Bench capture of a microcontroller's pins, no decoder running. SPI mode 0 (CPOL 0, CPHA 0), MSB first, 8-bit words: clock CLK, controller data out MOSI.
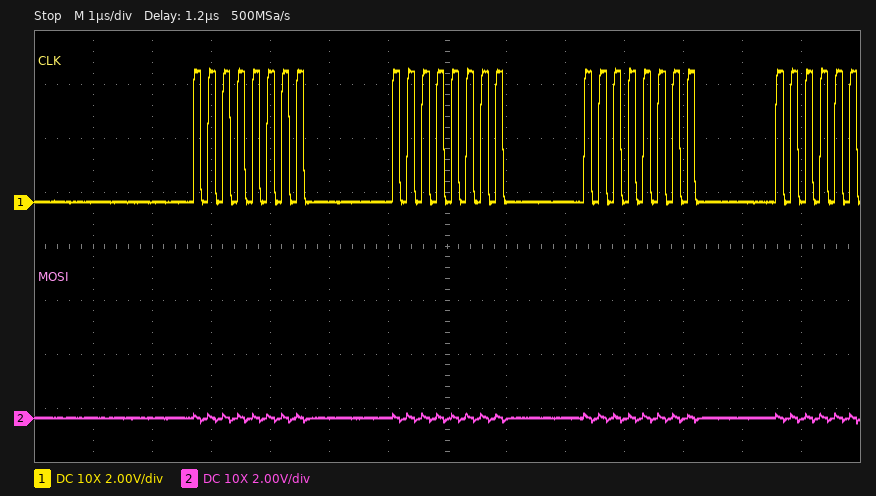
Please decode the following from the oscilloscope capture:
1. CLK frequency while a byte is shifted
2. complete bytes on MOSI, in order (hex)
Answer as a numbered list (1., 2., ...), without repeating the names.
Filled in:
1. 4 MHz
2. 00 00 00
